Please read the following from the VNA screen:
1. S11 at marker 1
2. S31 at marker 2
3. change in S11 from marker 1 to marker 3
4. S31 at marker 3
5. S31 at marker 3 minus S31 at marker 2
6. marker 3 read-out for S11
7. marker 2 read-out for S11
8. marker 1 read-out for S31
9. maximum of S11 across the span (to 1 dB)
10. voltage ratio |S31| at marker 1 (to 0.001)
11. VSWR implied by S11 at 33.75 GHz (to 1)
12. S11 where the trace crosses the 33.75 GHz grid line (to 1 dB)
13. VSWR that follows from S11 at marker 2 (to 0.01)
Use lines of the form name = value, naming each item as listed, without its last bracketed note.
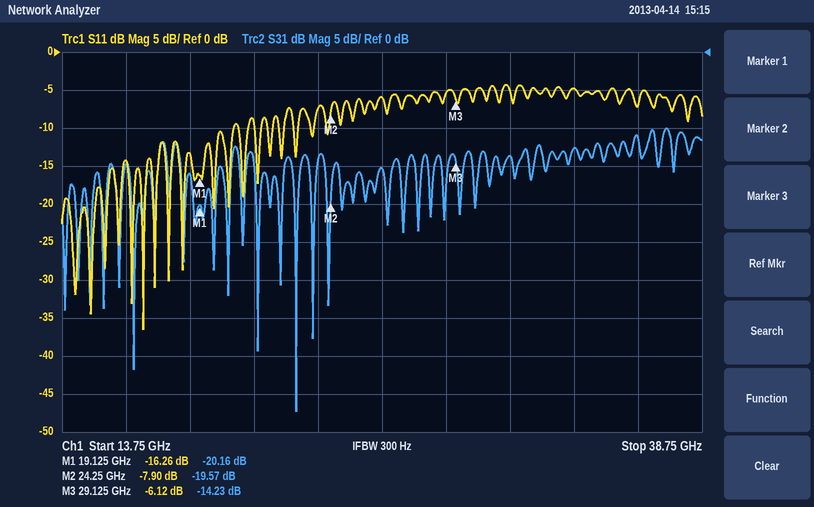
S11 at marker 1 = -16.26 dB
S31 at marker 2 = -19.57 dB
change in S11 from marker 1 to marker 3 = 10.14 dB
S31 at marker 3 = -14.23 dB
S31 at marker 3 minus S31 at marker 2 = 5.34 dB
marker 3 read-out for S11 = -6.12 dB
marker 2 read-out for S11 = -7.90 dB
marker 1 read-out for S31 = -20.16 dB
maximum of S11 across the span = -4 dB
voltage ratio |S31| at marker 1 = 0.098
VSWR implied by S11 at 33.75 GHz = 4
S11 where the trace crosses the 33.75 GHz grid line = -5 dB
VSWR that follows from S11 at marker 2 = 2.35
